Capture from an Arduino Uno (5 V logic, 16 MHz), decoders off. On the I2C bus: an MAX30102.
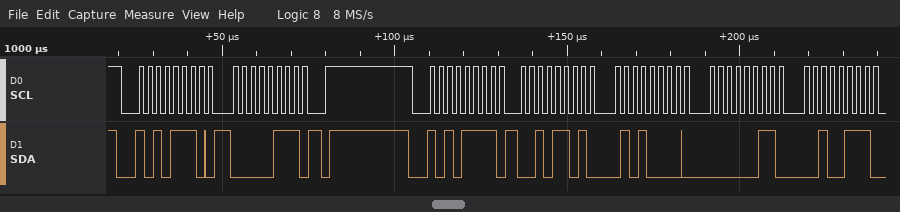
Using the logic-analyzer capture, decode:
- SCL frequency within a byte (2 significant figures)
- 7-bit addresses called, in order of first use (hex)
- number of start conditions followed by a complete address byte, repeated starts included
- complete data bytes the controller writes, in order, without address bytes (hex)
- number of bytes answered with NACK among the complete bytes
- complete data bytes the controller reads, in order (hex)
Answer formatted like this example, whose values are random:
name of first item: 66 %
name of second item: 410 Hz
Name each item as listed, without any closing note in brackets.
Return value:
SCL frequency within a byte: 400 kHz
7-bit addresses called, in order of first use: 0x57
number of start conditions followed by a complete address byte, repeated starts included: 2
complete data bytes the controller writes, in order, without address bytes: 07
number of bytes answered with NACK among the complete bytes: 0
complete data bytes the controller reads, in order: 2D 50 03 27
